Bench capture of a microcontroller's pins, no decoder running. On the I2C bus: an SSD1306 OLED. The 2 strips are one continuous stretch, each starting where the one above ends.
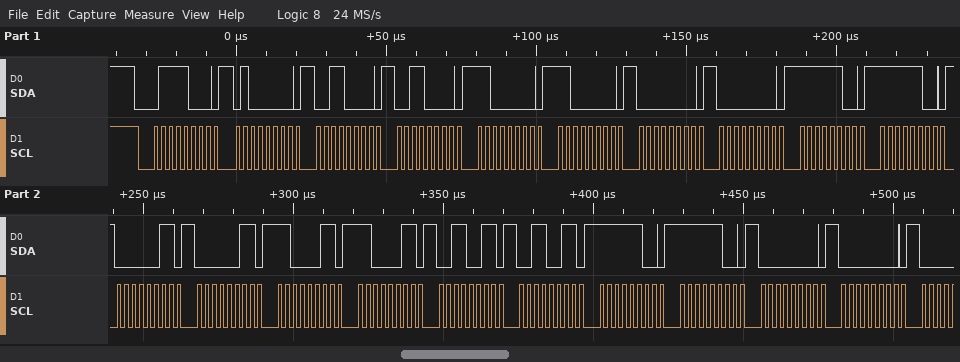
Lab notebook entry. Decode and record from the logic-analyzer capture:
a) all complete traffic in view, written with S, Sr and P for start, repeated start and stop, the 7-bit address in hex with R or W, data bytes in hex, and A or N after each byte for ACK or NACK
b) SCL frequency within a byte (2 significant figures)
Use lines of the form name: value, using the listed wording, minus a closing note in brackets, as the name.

all complete traffic in view, written with S, Sr and P for start, repeated start and stop, the 7-bit address in hex with R or W, data bytes in hex, and A or N after each byte for ACK or NACK: S 3CW A 40 A 30 A 30 A C0 A C0 A 00 A 00 A FC A FC A 03 A 03 A C3 A C3 A 33 A 33 A FC A FC A 00 A 00 A
SCL frequency within a byte: 400 kHz
